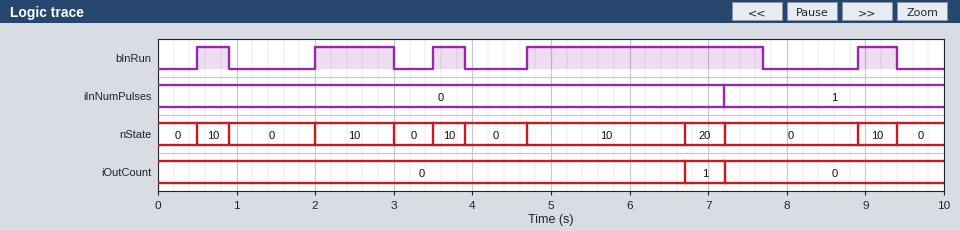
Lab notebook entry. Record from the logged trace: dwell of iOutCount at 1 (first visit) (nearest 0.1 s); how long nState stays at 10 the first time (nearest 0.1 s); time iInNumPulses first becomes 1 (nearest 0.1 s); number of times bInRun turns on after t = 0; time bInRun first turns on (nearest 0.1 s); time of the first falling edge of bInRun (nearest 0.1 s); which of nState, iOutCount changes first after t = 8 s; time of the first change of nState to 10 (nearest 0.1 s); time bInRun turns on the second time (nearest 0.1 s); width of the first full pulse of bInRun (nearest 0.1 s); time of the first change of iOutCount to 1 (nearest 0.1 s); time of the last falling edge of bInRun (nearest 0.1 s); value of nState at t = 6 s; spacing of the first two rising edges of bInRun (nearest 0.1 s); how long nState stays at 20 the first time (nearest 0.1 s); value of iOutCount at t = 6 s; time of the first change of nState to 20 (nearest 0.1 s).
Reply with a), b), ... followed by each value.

a) 0.5 s
b) 0.4 s
c) 7.2 s
d) 5
e) 0.5 s
f) 0.9 s
g) nState
h) 0.5 s
i) 2.0 s
j) 0.4 s
k) 6.7 s
l) 9.4 s
m) 10
n) 1.5 s
o) 0.5 s
p) 0
q) 6.7 s
